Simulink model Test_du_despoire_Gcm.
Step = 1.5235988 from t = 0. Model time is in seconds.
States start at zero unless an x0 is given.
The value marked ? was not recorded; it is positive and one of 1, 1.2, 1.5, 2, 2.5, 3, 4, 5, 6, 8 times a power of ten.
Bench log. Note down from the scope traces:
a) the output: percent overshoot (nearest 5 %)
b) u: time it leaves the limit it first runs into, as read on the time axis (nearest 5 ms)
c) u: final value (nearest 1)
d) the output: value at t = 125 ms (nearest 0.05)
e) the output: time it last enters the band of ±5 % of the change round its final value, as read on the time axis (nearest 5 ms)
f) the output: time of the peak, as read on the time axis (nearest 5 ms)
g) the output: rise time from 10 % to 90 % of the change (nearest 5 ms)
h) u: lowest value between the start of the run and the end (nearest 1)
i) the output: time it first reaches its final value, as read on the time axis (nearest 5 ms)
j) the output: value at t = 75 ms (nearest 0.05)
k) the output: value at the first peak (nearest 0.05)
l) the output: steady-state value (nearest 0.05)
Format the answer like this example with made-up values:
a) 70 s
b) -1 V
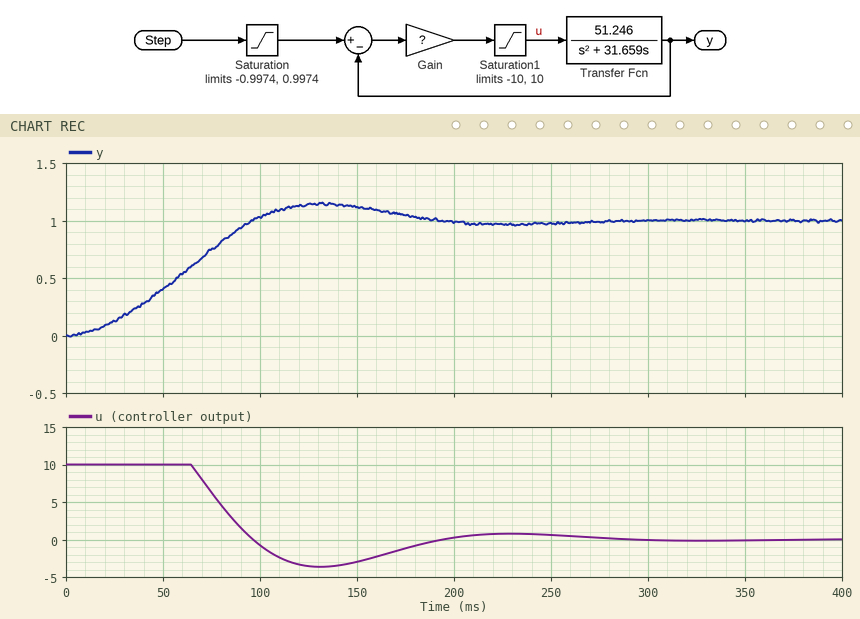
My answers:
a) 15 %
b) 65 ms
c) 0
d) 1.15
e) 175 ms
f) 130 ms
g) 65 ms
h) -4
i) 95 ms
j) 0.75
k) 1.15
l) 1.00
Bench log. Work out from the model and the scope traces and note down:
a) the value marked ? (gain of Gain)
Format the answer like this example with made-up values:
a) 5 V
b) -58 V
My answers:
a) 25
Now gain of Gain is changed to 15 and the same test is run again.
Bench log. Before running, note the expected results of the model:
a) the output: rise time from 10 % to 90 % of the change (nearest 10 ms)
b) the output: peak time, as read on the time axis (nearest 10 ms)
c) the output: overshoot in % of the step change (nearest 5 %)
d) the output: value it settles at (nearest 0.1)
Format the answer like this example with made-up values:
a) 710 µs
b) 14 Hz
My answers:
a) 70 ms
b) 150 ms
c) 10 %
d) 1.0
